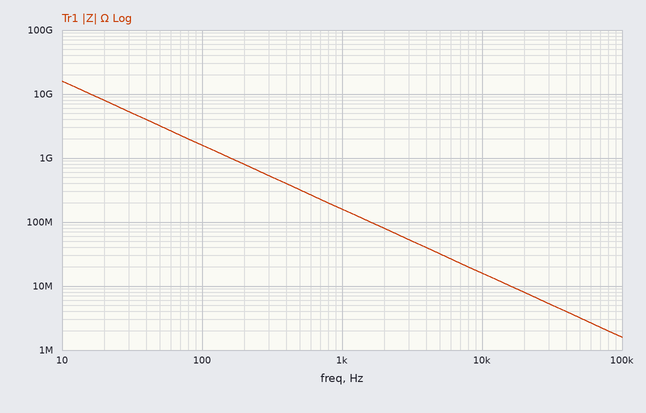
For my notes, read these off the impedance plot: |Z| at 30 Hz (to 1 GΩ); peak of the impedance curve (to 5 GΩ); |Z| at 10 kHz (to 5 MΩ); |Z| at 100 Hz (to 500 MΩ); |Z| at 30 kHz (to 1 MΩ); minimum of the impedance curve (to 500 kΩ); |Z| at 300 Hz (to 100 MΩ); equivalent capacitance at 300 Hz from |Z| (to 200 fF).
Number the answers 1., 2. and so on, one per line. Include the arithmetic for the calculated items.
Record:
1. 5 GΩ
2. 15 GΩ
3. 15 MΩ
4. 1.5 GΩ
5. 5 MΩ
6. 1.5 MΩ
7. 500 MΩ
8. C = 1/(2π × 300 Hz × 500 MΩ) ≈ 1.06 pF, so 1.0 pF to the nearest 200 fF
